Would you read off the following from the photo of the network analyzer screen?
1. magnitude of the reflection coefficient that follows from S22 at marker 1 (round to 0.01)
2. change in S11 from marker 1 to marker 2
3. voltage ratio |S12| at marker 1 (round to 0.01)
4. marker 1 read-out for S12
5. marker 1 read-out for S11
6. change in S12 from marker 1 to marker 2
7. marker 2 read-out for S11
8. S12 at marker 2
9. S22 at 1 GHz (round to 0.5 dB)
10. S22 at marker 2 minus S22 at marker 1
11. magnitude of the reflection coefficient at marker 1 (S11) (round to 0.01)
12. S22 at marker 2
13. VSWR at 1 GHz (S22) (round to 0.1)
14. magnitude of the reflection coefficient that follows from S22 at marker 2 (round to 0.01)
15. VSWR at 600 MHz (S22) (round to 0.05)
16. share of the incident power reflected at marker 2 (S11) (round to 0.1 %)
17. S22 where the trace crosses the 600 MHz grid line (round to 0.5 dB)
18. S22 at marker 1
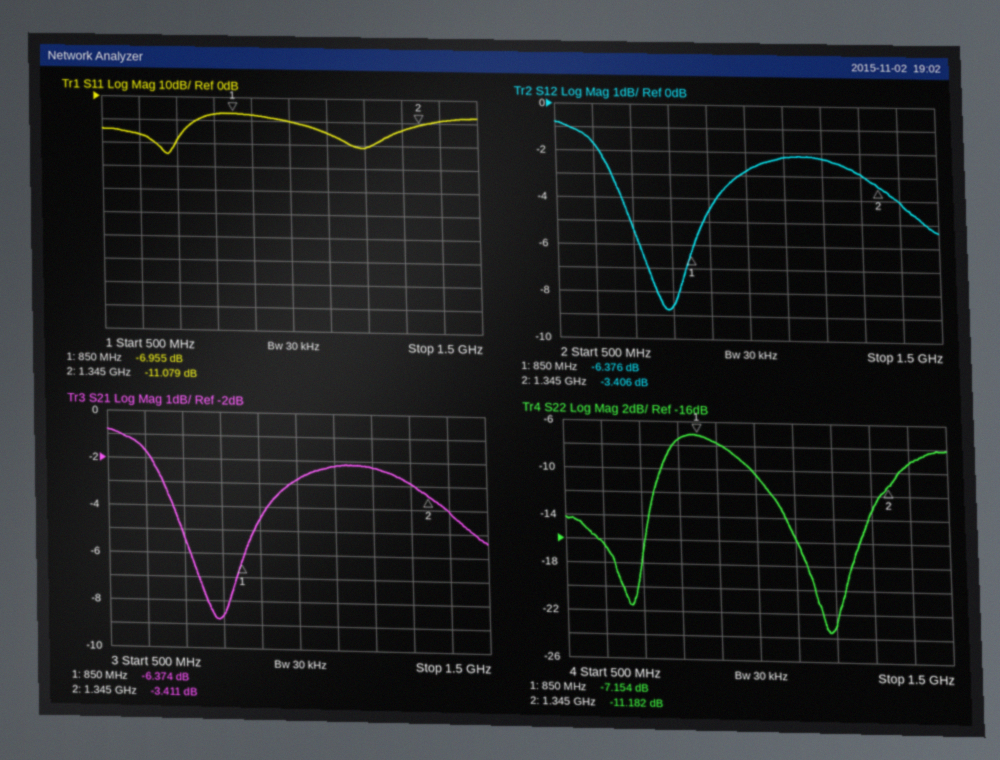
0.44
-4.124 dB
0.48
-6.376 dB
-6.955 dB
2.970 dB
-11.079 dB
-3.406 dB
-10.5 dB
-4.028 dB
0.45
-11.182 dB
1.9
0.28
1.35
7.8 %
-16.5 dB
-7.154 dB
